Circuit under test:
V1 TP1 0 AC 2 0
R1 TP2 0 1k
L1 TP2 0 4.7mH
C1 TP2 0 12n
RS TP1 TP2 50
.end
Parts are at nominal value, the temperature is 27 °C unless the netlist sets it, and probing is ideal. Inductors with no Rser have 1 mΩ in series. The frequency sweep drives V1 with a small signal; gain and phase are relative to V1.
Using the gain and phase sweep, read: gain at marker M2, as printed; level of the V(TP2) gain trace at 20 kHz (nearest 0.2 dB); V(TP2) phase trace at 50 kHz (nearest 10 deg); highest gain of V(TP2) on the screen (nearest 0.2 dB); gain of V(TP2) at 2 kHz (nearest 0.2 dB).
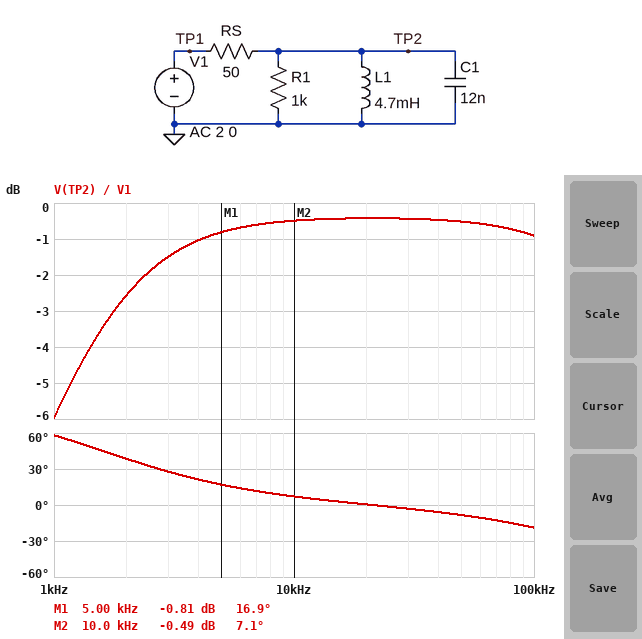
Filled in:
-0.49 dB
-0.4 dB
-10 deg
-0.4 dB
-2.6 dB
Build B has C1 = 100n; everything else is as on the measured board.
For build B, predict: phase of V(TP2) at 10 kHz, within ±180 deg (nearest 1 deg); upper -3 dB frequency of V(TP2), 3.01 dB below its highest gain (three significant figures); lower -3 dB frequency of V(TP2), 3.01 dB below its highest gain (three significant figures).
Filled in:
-8 deg
35.0 kHz
1.54 kHz
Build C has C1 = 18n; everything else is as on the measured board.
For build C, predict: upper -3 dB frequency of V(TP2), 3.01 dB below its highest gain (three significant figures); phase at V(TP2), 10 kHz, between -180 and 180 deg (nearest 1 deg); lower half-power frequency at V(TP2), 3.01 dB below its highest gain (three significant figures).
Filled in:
187 kHz
6 deg
1.60 kHz
